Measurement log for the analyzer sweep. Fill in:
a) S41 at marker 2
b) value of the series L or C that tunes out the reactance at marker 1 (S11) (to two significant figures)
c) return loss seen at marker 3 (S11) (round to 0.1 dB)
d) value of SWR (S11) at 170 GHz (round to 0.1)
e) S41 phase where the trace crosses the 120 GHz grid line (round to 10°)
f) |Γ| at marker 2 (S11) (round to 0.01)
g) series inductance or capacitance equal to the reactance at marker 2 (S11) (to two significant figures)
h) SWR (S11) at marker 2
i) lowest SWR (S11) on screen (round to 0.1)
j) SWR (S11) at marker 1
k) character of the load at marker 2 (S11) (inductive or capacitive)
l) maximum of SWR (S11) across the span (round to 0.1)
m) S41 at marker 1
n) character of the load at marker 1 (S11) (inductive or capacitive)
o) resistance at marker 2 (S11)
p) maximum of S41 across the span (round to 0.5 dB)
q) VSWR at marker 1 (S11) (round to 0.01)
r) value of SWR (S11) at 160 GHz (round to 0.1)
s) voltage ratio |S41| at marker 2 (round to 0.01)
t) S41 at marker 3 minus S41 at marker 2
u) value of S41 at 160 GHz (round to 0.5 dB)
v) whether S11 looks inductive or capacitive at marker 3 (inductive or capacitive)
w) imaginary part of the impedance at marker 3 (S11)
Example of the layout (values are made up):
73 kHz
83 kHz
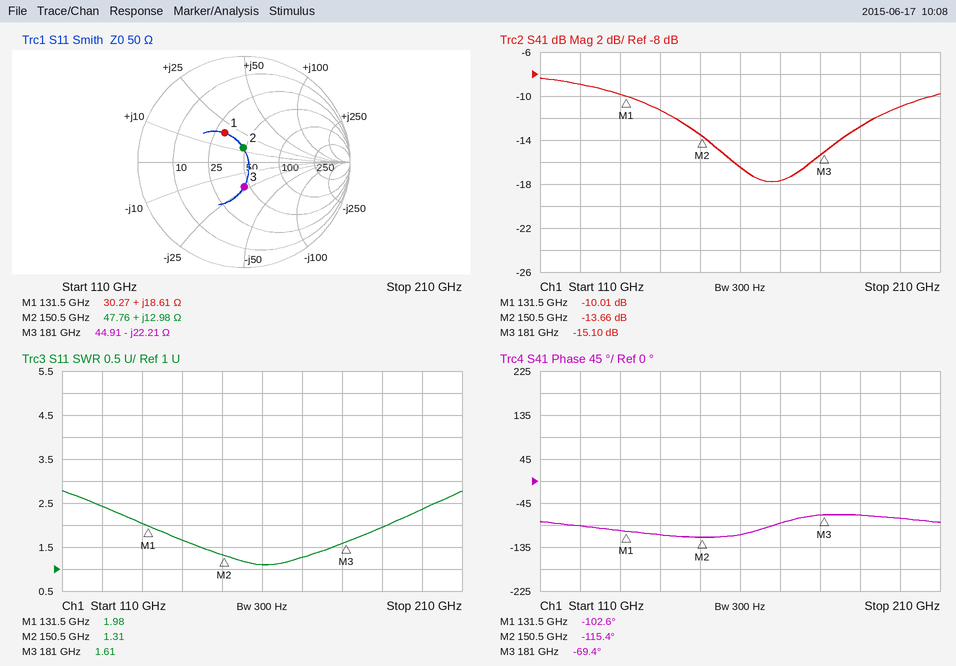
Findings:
-13.66 dB
65 fF
12.6 dB
1.3
-90°
0.13
14 pH
1.31
1.1
1.98
inductive
2.8
-10.01 dB
inductive
47.76 Ω
-8.5 dB
1.98
1.1
0.21
-1.44 dB
-16.5 dB
capacitive
-22.21 Ω
